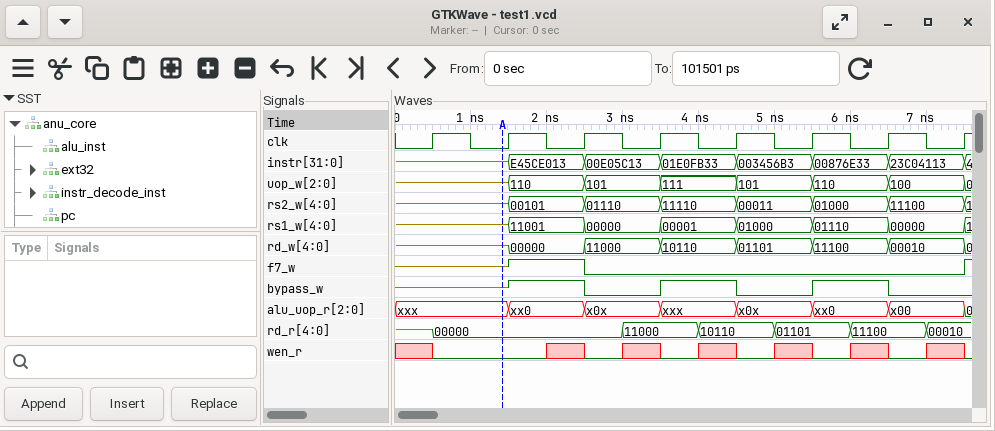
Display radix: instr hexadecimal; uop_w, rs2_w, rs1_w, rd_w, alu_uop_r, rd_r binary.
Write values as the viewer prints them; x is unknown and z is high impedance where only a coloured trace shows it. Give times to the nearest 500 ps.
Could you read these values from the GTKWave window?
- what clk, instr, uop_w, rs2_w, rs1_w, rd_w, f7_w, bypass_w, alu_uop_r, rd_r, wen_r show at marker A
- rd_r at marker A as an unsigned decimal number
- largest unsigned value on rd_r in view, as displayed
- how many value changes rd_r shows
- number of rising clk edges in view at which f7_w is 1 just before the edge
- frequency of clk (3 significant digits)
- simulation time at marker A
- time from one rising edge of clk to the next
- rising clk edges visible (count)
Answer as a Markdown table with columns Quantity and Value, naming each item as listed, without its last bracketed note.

| Quantity | Value |
|---|---|
| what clk, instr, uop_w, rs2_w, rs1_w, rd_w, f7_w, bypass_w, alu_uop_r, rd_r, wen_r show at marker A | clk=0, instr=z, uop_w=z, rs2_w=z, rs1_w=z, rd_w=z, f7_w=z, bypass_w=z, alu_uop_r=xxx, rd_r=00000, wen_r=0 |
| rd_r at marker A as an unsigned decimal number | 0 |
| largest unsigned value on rd_r in view, as displayed | 11100 |
| how many value changes rd_r shows | 6 |
| number of rising clk edges in view at which f7_w is 1 just before the edge | 1 |
| frequency of clk | 1.00 GHz |
| simulation time at marker A | 1500 ps |
| time from one rising edge of clk to the next | 1000 ps |
| rising clk edges visible | 8 |
